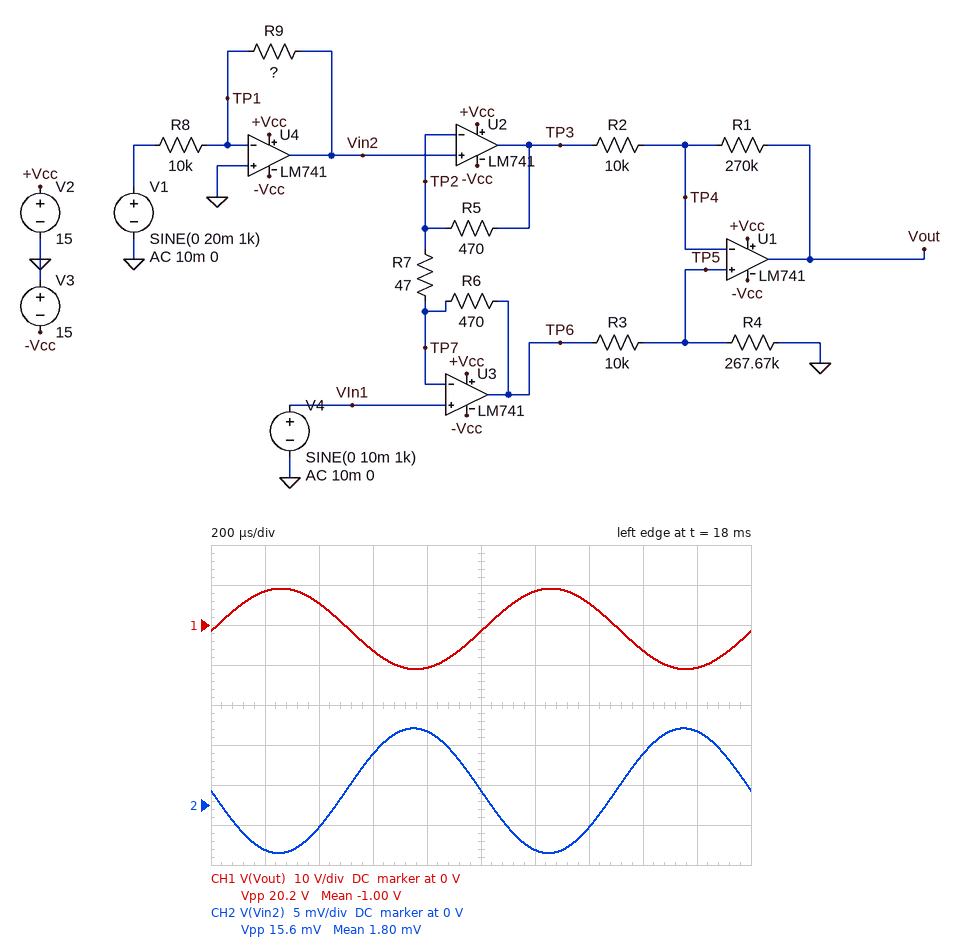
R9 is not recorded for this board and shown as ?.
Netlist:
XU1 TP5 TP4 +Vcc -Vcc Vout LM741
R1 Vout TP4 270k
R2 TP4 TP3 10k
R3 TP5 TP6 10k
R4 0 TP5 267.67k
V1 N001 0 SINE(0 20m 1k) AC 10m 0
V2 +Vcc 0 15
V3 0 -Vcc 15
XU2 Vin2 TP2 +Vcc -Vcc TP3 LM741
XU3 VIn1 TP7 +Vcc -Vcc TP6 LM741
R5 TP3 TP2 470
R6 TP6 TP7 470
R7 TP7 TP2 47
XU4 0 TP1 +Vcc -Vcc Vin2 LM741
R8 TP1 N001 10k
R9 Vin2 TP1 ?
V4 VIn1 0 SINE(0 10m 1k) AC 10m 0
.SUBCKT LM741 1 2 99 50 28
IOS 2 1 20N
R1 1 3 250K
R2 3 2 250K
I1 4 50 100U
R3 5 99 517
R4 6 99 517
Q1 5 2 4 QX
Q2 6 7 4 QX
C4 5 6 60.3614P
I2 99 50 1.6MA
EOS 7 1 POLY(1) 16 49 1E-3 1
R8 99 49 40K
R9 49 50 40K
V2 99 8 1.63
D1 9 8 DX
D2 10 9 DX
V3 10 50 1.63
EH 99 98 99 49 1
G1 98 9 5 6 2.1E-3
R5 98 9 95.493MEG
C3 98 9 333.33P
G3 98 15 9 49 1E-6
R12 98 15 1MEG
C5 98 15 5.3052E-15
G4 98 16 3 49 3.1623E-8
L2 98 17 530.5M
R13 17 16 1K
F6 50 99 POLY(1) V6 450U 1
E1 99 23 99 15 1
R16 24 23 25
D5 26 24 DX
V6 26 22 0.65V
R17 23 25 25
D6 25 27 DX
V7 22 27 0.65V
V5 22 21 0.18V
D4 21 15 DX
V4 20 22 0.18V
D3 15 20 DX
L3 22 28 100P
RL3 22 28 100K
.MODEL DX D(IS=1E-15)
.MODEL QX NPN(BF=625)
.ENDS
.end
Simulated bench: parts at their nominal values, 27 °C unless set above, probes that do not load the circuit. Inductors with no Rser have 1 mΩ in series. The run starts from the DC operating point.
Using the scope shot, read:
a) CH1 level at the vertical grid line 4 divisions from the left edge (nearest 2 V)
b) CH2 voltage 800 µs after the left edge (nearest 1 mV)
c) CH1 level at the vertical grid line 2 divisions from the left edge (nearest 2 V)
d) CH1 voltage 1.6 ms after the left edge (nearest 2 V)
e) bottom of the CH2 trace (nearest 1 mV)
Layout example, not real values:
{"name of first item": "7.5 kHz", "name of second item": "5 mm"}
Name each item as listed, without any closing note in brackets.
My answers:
{"CH1 level at the vertical grid line 4 divisions from the left edge": "-10 V", "CH2 voltage 800 µs after the left edge": "9 mV", "CH1 level at the vertical grid line 2 divisions from the left edge": "6 V", "CH1 voltage 1.6 ms after the left edge": "-6 V", "bottom of the CH2 trace": "-6 mV"}
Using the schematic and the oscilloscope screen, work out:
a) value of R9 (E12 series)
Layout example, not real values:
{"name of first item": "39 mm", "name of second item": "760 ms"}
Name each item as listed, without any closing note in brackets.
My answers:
{"value of R9": "3.9 kΩ"}
